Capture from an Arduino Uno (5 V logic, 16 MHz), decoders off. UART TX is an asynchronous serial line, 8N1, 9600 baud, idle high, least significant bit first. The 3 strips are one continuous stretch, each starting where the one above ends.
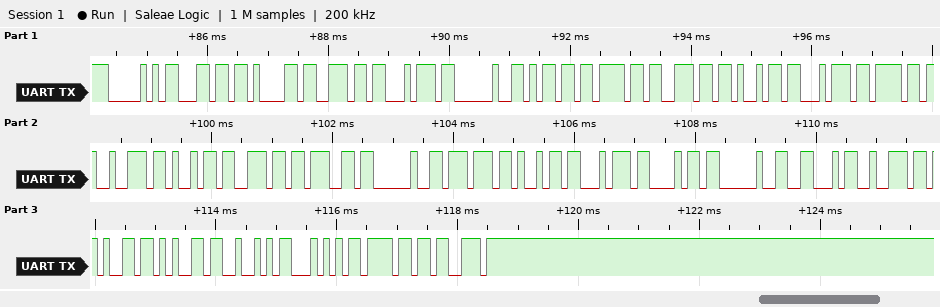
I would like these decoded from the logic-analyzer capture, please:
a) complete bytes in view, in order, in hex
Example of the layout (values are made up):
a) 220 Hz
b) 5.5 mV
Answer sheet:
a) 50 6C 61 6E 74 20 6D 6F 6E 69 74 6F 72 69 6E 67 20 77 69 74 68 20 46 72 65 65 52 54 6F 73
